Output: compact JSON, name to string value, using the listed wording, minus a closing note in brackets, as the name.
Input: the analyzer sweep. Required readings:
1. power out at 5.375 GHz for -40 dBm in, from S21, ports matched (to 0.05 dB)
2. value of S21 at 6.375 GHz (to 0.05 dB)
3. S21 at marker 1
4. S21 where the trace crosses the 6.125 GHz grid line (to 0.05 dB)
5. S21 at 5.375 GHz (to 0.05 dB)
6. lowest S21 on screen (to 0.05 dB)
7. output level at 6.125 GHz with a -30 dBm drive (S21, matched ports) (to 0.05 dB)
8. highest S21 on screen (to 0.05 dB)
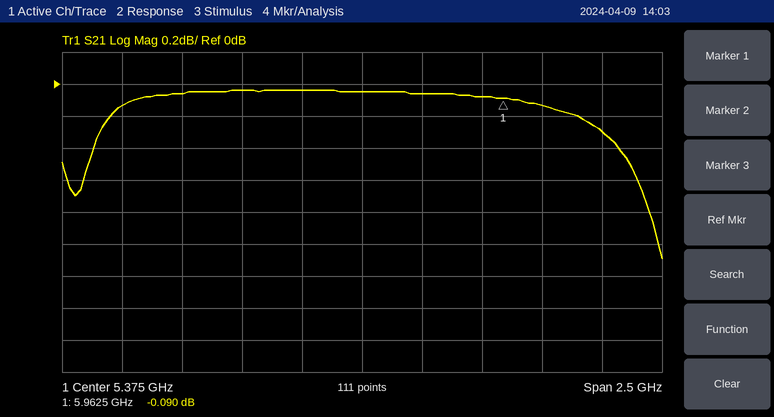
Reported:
{"power out at 5.375 GHz for -40 dBm in, from S21, ports matched": "-40.05 dBm", "value of S21 at 6.375 GHz": "-0.30 dB", "S21 at marker 1": "-0.090 dB", "S21 where the trace crosses the 6.125 GHz grid line": "-0.15 dB", "S21 at 5.375 GHz": "-0.05 dB", "lowest S21 on screen": "-1.10 dB", "output level at 6.125 GHz with a -30 dBm drive (S21, matched ports)": "-30.15 dBm", "highest S21 on screen": "-0.05 dB"}
